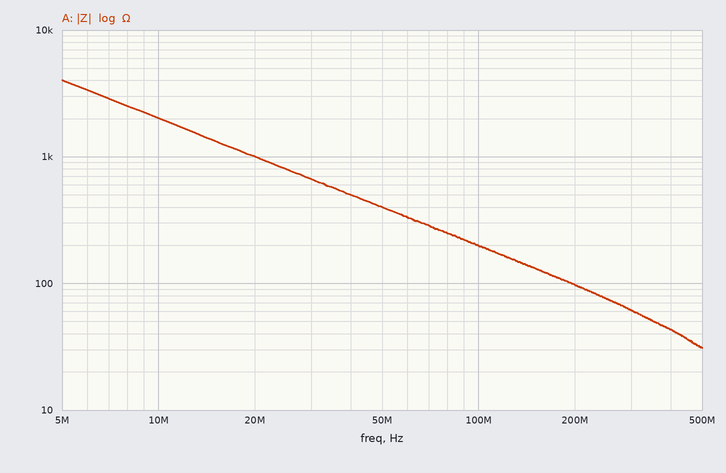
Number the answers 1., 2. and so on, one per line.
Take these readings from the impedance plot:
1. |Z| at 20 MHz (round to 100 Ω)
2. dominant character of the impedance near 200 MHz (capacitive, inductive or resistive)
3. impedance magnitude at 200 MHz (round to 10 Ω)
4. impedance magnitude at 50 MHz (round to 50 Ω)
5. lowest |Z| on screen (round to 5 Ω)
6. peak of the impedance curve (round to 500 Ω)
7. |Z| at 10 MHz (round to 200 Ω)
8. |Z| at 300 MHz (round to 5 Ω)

1. 1.0 kΩ
2. capacitive
3. 100 Ω
4. 400 Ω
5. 30 Ω
6. 4.0 kΩ
7. 2.0 kΩ
8. 60 Ω
